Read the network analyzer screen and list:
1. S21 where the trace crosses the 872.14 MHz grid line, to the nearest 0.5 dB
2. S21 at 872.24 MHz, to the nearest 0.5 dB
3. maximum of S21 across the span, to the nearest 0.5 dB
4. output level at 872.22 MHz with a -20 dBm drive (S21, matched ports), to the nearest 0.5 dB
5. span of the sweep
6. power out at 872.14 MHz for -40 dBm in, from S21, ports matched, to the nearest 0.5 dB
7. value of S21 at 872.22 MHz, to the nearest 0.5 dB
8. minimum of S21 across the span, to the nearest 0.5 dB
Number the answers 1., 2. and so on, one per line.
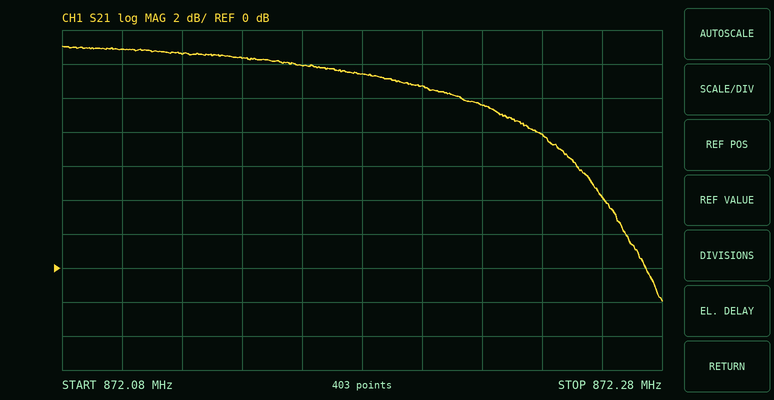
1. 12.5 dB
2. 8.0 dB
3. 13.0 dB
4. -10.5 dBm
5. 200 kHz
6. -27.5 dBm
7. 9.5 dB
8. -2.0 dB
